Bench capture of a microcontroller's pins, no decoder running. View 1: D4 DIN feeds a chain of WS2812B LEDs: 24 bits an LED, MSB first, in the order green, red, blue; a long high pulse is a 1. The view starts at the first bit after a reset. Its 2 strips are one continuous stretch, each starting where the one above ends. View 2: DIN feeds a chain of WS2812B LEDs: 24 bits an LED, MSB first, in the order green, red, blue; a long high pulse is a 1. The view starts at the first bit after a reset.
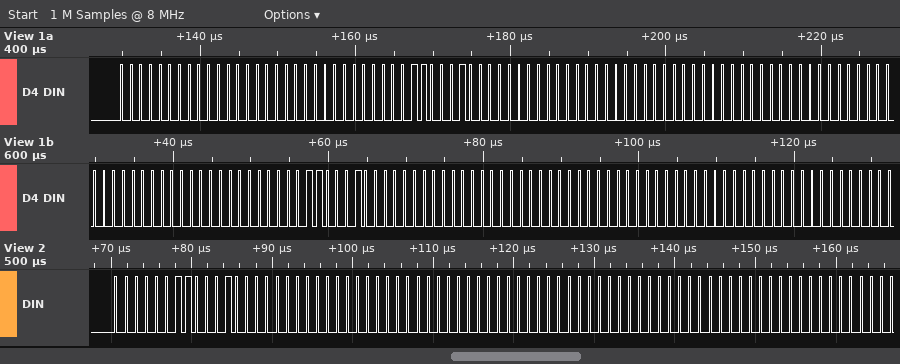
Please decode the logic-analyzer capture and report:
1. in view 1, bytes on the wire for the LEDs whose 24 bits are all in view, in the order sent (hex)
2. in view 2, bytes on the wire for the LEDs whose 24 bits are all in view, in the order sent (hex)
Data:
00 00 00 03 10 00 00 00 00 00 00 00 03 10 00 00 00 00
03 10 00 00 00 00 00 00 00
